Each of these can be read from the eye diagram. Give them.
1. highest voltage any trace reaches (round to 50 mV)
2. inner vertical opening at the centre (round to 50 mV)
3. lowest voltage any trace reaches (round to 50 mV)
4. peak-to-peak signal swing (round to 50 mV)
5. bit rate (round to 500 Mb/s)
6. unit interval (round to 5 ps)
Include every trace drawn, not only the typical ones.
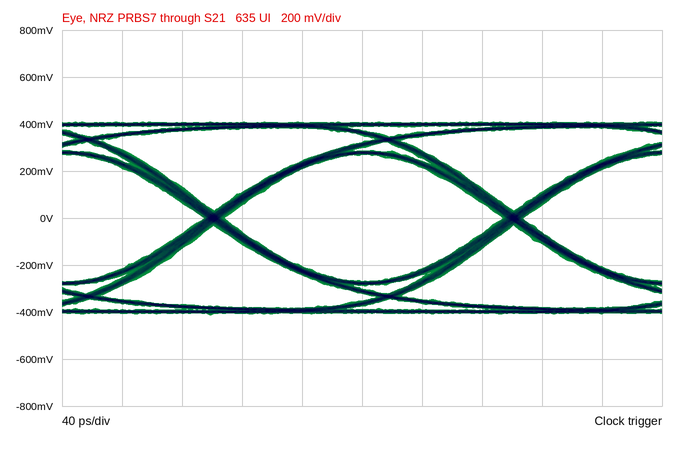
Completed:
400 mV
550 mV
-400 mV
800 mV
5.0 Gb/s
200 ps
